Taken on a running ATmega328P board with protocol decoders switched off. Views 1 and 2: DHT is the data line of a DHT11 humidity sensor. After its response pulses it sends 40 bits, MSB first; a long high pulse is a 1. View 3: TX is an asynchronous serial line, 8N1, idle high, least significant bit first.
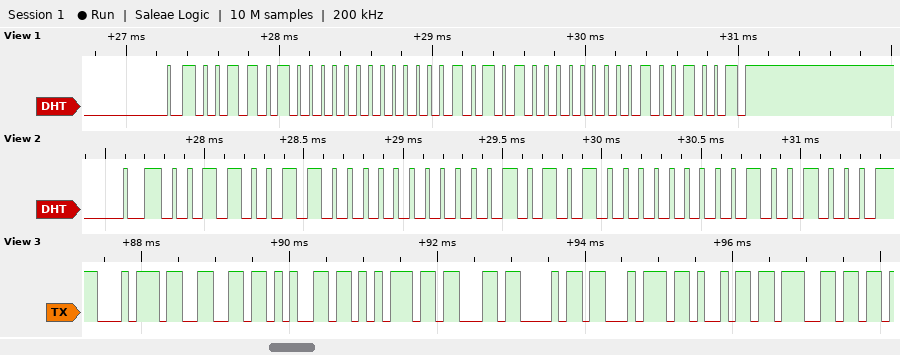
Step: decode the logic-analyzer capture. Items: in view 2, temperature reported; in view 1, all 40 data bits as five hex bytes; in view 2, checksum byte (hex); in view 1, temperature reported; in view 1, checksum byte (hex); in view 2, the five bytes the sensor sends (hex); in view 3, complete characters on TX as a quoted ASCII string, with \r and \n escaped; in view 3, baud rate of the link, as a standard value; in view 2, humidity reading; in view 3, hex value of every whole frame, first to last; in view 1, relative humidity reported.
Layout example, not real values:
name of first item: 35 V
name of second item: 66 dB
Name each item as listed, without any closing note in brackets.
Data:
in view 2, temperature reported: 21.0 °C
in view 1, all 40 data bits as five hex bytes: 34 00 15 00 49
in view 2, checksum byte: 0x48
in view 1, temperature reported: 21.0 °C
in view 1, checksum byte: 0x49
in view 2, the five bytes the sensor sends: 33 00 15 00 48
in view 3, complete characters on TX as a quoted ASCII string, with \r and \n escaped: "tfeuchtig"
in view 3, baud rate of the link, as a standard value: 9600 baud
in view 2, humidity reading: 51 %
in view 3, hex value of every whole frame, first to last: 0x74 0x66 0x65 0x75 0x63 0x68 0x74 0x69 0x67
in view 1, relative humidity reported: 52 %
